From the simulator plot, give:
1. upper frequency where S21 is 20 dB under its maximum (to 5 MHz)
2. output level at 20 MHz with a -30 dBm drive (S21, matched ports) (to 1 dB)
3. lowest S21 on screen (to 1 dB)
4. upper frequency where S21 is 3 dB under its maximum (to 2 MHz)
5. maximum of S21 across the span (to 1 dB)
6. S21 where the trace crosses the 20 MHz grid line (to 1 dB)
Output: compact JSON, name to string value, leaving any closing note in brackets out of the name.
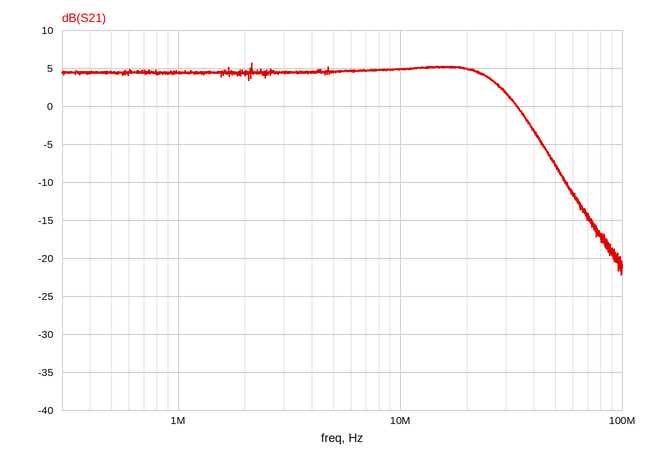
{"upper frequency where S21 is 20 dB under its maximum": "70 MHz", "output level at 20 MHz with a -30 dBm drive (S21, matched ports)": "-25 dBm", "lowest S21 on screen": "-22 dB", "upper frequency where S21 is 3 dB under its maximum": "28 MHz", "maximum of S21 across the span": "6 dB", "S21 where the trace crosses the 20 MHz grid line": "5 dB"}
